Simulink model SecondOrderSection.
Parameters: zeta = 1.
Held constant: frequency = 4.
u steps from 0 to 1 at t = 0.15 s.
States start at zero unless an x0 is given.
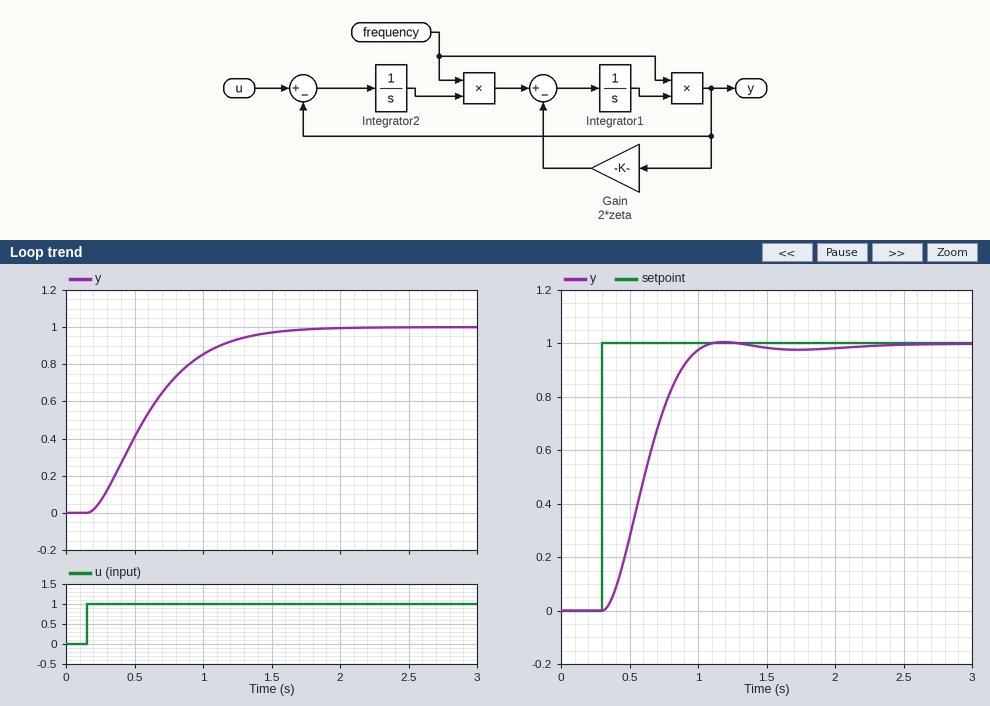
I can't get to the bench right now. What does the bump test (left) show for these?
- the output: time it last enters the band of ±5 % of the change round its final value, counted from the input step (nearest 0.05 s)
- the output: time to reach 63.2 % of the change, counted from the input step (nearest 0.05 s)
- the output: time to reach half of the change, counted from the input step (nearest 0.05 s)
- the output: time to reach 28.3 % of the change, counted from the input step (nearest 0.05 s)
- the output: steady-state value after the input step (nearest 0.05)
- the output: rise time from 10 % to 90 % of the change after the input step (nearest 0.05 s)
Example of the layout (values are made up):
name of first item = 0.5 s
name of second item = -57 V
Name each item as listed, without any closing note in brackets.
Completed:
the output: time it last enters the band of ±5 % of the change round its final value, counted from the input step = 1.20 s
the output: time to reach 63.2 % of the change, counted from the input step = 0.55 s
the output: time to reach half of the change, counted from the input step = 0.40 s
the output: time to reach 28.3 % of the change, counted from the input step = 0.25 s
the output: steady-state value after the input step = 1.00
the output: rise time from 10 % to 90 % of the change after the input step = 0.85 s
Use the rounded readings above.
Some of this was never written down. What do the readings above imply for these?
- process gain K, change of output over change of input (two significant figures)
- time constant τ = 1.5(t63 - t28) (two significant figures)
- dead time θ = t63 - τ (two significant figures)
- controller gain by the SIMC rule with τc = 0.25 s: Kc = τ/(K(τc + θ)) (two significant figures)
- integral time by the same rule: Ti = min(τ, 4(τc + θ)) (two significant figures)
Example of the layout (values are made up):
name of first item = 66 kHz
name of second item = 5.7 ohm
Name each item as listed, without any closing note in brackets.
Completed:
process gain K, change of output over change of input = 1.0
time constant τ = 1.5(t63 - t28) = 0.45 s
dead time θ = t63 - τ = 0.10 s
controller gain by the SIMC rule with τc = 0.25 s: Kc = τ/(K(τc + θ)) = 1.3
integral time by the same rule: Ti = min(τ, 4(τc + θ)) = 0.45 s
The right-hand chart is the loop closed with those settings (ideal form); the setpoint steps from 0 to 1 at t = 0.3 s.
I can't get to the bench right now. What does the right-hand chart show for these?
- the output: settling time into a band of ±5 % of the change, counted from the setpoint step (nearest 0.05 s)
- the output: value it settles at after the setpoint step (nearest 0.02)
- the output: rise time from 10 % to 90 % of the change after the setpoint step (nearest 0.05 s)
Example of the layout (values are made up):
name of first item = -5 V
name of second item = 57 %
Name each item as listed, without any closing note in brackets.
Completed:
the output: settling time into a band of ±5 % of the change, counted from the setpoint step = 0.65 s
the output: value it settles at after the setpoint step = 1.00
the output: rise time from 10 % to 90 % of the change after the setpoint step = 0.45 s
